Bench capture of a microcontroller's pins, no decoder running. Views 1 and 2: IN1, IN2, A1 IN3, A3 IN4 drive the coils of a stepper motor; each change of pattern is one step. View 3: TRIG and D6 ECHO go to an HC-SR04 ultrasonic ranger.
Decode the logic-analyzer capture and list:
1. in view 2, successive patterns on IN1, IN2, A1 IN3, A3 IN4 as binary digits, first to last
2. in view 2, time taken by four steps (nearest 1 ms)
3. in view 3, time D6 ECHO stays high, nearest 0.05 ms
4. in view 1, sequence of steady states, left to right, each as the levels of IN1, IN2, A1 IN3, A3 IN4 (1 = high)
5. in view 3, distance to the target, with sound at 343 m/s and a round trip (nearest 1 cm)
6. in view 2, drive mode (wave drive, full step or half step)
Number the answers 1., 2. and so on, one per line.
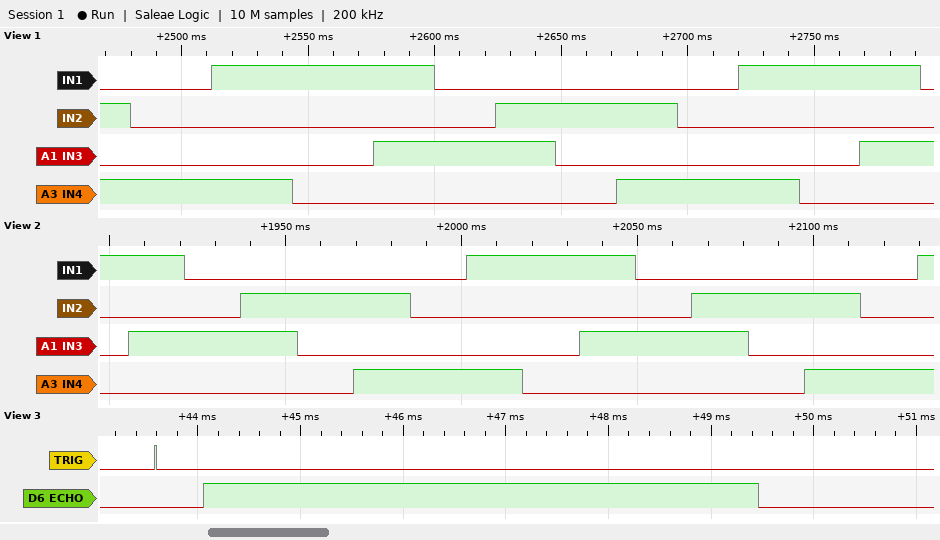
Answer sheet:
1. 1000 1010 0010 0110 0100 0101 0001 1001 1000 1010 0010 0110 0100 0101 0001 1001
2. 64 ms
3. 5.40 ms
4. 0101 0001 1001 1000 1010 0010 0110 0100 0101 0001 1001 1000 1010 0010
5. 93 cm
6. half step
